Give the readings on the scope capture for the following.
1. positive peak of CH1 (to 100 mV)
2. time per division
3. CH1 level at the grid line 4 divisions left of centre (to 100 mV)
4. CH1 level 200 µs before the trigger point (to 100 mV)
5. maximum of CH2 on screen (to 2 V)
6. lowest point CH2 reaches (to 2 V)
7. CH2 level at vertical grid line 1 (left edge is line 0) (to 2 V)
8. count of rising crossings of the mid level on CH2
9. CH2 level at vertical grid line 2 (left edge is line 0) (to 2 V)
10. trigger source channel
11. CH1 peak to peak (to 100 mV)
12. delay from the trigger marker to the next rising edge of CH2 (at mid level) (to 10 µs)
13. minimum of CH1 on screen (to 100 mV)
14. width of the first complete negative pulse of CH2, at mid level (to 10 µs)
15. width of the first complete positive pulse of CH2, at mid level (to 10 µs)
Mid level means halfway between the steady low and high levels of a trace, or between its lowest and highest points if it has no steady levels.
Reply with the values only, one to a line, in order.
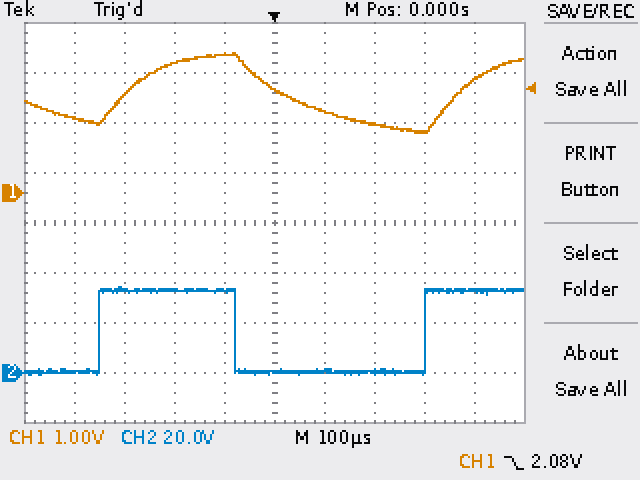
2.8 V
100 µs
1.5 V
2.6 V
34 V
0 V
0 V
2
34 V
CH1
1.6 V
300 µs
1.2 V
380 µs
270 µs
